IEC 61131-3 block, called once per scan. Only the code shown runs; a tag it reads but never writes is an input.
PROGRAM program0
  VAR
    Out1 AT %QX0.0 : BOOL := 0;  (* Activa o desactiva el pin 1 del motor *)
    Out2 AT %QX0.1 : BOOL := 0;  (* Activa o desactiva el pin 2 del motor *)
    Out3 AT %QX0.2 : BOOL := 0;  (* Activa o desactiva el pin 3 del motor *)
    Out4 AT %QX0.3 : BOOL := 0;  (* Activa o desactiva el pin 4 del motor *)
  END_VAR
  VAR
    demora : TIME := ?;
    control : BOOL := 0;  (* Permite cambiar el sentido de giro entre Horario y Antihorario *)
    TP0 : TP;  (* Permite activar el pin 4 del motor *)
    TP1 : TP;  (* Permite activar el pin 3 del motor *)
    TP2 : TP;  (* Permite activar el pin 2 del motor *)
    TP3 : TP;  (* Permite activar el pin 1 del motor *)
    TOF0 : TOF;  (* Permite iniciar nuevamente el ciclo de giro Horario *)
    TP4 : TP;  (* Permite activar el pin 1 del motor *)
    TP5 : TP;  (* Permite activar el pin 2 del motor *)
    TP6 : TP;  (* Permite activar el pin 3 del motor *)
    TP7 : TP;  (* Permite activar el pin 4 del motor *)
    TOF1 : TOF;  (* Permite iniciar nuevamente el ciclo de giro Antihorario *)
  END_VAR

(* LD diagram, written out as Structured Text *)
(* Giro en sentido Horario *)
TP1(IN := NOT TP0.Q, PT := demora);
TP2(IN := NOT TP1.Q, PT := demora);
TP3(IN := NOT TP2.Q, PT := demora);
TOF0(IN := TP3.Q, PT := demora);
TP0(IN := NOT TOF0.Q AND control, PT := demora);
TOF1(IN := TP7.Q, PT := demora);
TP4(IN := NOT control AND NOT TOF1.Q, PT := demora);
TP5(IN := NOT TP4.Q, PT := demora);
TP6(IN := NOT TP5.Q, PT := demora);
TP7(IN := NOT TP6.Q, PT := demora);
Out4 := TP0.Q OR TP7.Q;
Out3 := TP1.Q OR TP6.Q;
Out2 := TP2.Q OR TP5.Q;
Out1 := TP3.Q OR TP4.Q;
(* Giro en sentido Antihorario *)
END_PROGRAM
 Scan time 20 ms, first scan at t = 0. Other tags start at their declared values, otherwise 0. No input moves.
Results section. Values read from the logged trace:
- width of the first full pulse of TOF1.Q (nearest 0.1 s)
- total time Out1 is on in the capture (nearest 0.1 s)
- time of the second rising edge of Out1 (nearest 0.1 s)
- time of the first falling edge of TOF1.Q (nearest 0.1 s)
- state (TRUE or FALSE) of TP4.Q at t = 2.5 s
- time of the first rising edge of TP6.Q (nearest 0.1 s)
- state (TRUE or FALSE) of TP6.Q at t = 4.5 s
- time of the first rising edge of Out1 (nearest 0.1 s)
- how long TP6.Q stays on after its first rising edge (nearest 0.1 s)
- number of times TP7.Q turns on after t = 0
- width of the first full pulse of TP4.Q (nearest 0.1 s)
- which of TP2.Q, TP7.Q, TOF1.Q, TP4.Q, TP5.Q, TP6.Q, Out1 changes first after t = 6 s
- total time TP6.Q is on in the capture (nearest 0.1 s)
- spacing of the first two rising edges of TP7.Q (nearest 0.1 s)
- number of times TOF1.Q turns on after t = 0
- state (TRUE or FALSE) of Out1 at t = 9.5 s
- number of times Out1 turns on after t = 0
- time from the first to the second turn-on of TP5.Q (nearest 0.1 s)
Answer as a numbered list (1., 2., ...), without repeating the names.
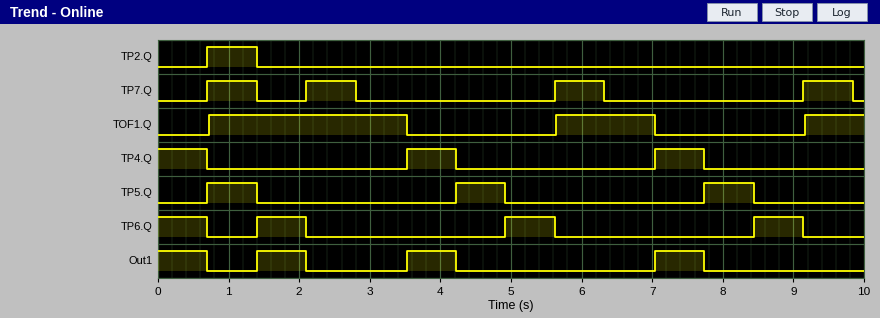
1. 2.8 s
2. 2.8 s
3. 3.5 s
4. 3.5 s
5. FALSE
6. 1.4 s
7. FALSE
8. 1.4 s
9. 0.7 s
10. 4
11. 0.7 s
12. TP7.Q
13. 2.8 s
14. 1.4 s
15. 3
16. FALSE
17. 3
18. 3.5 s
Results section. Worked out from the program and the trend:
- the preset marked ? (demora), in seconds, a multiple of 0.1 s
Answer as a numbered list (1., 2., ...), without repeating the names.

1. 0.7 s
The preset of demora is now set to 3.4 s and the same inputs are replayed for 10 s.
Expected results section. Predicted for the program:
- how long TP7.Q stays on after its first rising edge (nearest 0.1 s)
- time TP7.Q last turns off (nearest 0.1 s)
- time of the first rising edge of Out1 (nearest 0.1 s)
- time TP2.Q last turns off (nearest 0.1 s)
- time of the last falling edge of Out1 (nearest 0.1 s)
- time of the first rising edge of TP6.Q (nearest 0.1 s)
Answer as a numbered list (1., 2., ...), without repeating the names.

1. 3.4 s
2. 6.8 s
3. 6.8 s
4. 6.8 s
5. 3.4 s
6. 6.8 s
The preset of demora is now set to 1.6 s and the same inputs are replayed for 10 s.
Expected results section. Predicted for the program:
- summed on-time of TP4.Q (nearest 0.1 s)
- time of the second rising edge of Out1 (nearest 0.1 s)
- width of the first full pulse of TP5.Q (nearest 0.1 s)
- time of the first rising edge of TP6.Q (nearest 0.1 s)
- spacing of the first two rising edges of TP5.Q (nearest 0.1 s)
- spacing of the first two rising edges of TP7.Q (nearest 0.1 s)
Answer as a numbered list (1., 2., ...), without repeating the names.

1. 3.2 s
2. 8.0 s
3. 1.6 s
4. 3.2 s
5. 8.0 s
6. 3.2 s
